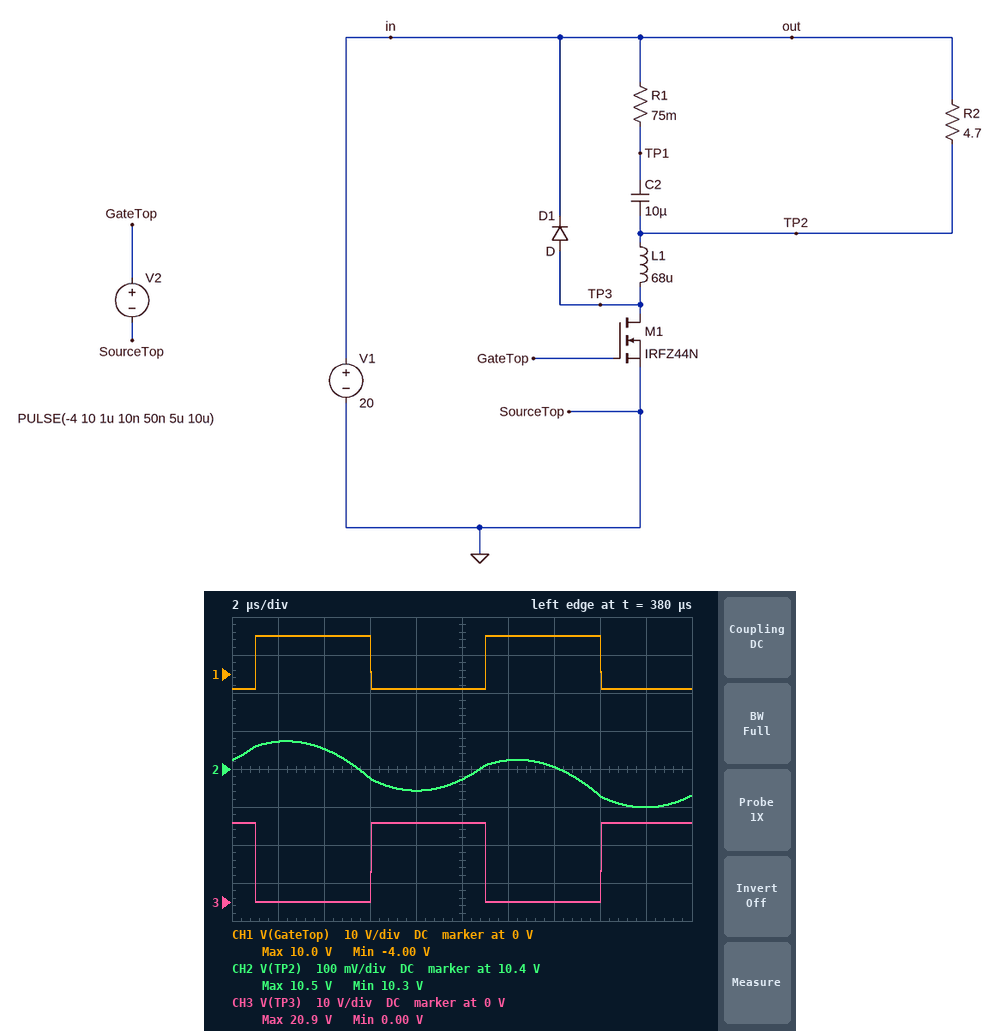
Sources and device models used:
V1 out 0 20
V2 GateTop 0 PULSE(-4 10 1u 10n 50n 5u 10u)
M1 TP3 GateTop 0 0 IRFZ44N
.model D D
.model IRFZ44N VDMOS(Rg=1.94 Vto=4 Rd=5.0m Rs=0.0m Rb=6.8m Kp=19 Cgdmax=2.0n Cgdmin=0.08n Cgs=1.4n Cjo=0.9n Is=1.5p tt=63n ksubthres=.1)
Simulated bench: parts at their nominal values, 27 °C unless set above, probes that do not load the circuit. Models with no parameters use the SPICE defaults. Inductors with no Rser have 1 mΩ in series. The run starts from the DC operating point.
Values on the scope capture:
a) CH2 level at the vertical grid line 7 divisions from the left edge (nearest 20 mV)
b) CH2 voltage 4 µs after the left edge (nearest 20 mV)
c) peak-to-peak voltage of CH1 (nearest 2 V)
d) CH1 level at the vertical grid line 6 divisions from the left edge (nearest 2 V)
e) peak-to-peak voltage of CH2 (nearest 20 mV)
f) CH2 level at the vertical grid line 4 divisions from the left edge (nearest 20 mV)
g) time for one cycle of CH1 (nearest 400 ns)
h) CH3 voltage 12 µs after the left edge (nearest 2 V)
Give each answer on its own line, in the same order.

10.40 V
10.46 V
14 V
10 V
180 mV
10.34 V
10.0 µs
0 V
